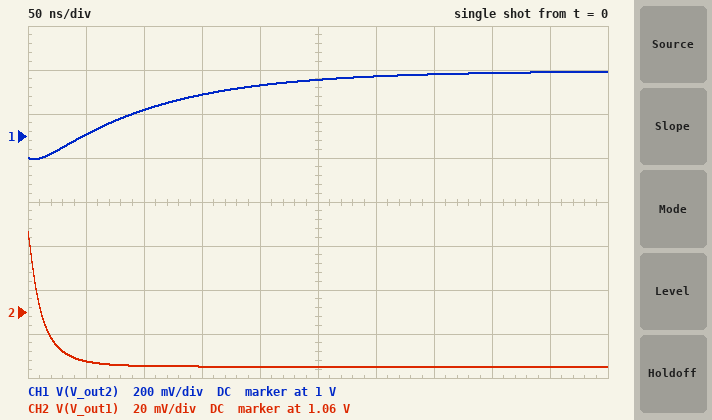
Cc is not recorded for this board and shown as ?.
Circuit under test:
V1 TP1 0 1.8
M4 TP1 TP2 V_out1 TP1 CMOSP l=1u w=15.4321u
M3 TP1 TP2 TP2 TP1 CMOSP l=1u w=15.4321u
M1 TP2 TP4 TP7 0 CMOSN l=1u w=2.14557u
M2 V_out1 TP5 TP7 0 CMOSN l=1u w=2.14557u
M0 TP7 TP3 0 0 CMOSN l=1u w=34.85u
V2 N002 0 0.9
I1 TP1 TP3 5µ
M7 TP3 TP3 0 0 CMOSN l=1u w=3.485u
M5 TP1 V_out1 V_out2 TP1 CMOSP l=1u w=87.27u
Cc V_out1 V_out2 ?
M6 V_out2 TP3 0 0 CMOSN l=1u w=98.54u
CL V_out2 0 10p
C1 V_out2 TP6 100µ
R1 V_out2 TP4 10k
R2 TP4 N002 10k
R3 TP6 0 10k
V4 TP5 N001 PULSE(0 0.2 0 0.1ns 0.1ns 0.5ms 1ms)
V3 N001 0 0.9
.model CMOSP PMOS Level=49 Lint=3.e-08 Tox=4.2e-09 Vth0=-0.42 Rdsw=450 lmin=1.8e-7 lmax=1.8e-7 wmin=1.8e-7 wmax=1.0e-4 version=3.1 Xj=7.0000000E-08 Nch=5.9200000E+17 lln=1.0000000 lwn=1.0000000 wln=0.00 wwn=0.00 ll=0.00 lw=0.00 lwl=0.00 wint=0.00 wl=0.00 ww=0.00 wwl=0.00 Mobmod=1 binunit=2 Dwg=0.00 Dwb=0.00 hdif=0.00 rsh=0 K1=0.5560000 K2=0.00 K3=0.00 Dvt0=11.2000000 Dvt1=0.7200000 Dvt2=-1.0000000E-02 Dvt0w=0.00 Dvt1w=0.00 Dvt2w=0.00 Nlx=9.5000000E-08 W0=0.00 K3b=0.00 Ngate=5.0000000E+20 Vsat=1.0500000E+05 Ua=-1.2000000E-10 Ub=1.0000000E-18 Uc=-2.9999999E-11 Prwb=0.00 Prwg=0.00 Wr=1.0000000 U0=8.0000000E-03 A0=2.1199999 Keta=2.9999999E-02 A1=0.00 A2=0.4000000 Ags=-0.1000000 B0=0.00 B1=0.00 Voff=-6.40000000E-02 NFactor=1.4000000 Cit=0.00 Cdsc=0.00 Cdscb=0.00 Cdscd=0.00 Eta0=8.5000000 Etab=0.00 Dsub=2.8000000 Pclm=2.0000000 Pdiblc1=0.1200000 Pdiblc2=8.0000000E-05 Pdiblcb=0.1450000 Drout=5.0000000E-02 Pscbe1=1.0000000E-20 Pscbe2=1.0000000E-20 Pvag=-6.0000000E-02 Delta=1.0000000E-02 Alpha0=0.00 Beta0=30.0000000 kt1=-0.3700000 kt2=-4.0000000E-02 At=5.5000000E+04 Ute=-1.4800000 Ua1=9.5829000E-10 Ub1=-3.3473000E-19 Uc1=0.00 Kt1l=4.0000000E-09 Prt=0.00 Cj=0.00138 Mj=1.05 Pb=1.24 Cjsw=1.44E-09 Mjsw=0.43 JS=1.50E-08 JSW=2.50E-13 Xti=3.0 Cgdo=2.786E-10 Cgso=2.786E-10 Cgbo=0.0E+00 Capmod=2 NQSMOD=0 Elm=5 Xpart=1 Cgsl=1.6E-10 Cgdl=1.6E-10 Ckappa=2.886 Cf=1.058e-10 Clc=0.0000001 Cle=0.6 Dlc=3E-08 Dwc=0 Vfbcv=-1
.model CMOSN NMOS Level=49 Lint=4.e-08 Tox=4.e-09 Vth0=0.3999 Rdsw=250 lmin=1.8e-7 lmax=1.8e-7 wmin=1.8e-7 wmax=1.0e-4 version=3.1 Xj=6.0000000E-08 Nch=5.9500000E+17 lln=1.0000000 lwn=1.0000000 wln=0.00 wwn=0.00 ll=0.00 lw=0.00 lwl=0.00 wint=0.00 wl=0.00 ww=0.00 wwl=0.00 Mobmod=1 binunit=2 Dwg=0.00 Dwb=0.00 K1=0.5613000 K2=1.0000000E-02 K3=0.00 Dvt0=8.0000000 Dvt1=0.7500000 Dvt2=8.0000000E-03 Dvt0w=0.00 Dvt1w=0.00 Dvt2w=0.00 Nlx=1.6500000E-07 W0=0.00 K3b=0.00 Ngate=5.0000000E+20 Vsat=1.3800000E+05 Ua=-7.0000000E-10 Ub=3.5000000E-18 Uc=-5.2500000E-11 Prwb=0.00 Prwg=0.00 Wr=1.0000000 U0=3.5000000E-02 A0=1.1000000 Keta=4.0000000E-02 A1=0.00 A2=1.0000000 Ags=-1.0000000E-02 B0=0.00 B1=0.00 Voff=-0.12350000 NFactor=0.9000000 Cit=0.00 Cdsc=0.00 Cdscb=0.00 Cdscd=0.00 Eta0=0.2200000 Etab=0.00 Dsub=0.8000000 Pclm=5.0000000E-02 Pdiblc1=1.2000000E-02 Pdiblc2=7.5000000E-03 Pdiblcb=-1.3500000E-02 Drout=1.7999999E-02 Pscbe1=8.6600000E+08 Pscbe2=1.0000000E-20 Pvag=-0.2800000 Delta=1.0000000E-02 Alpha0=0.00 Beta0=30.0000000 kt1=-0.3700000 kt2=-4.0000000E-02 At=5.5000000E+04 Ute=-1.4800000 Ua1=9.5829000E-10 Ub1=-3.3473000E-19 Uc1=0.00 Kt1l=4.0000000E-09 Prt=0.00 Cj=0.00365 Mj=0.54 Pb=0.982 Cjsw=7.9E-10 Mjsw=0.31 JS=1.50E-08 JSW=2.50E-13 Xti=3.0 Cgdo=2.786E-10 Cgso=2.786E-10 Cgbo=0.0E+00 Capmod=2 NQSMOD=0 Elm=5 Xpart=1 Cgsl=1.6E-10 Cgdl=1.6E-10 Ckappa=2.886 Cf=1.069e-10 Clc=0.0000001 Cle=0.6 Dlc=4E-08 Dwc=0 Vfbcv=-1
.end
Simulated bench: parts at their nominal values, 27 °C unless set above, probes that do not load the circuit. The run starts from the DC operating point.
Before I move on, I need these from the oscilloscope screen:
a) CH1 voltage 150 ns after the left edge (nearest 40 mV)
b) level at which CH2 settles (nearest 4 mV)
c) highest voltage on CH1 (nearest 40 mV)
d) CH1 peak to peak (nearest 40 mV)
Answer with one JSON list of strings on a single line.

["1.20 V", "1.036 V", "1.28 V", "400 mV"]
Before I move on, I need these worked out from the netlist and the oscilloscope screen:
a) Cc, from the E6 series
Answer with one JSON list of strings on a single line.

["6.8 pF"]
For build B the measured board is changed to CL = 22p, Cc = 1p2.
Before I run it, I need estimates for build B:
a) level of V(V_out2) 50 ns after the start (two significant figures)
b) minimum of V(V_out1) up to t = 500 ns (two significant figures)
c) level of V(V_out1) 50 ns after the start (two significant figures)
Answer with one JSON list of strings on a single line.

["1.3 V", "890 mV", "930 mV"]
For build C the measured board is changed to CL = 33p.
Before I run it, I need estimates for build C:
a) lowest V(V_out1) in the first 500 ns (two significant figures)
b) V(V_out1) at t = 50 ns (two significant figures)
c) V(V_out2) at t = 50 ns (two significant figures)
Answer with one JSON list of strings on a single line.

["990 mV", "1.0 V", "970 mV"]
